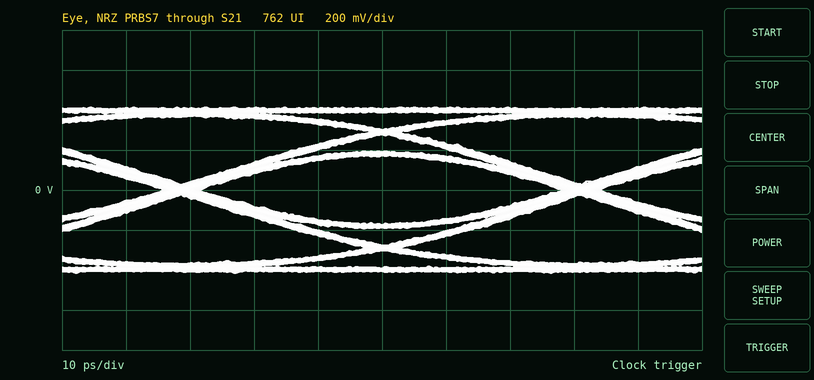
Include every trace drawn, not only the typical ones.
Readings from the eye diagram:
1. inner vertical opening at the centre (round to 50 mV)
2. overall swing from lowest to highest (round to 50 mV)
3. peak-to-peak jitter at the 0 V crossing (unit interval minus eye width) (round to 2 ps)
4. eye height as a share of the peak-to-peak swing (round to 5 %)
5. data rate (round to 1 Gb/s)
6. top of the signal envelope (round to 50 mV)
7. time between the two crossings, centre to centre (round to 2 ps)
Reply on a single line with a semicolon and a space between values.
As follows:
350 mV; 850 mV; 6 ps; 40 %; 16 Gb/s; 400 mV; 62 ps
